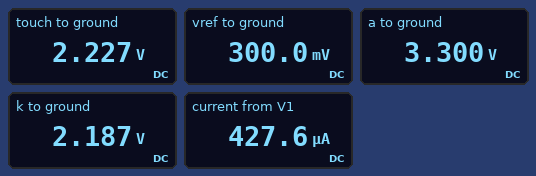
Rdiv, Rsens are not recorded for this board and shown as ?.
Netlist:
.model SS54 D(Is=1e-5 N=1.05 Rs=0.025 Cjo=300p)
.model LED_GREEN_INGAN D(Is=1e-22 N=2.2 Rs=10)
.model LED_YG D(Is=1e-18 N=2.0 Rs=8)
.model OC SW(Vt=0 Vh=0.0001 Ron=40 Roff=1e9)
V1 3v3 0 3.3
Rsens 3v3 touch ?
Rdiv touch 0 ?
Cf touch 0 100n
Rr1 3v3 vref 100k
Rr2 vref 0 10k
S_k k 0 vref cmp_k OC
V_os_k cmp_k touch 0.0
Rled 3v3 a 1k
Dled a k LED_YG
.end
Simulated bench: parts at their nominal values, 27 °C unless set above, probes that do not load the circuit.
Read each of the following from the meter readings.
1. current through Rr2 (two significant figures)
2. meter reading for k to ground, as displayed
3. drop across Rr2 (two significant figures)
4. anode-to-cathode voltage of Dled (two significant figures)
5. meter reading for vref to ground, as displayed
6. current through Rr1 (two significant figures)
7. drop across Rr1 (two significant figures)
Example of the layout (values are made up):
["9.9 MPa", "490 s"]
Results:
["30 µA", "2.187 V", "300 mV", "1.1 V", "300.0 mV", "30 µA", "3.0 V"]
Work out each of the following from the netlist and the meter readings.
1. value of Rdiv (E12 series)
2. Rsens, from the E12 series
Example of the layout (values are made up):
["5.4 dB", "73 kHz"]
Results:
["5.6 kΩ", "2.7 kΩ"]
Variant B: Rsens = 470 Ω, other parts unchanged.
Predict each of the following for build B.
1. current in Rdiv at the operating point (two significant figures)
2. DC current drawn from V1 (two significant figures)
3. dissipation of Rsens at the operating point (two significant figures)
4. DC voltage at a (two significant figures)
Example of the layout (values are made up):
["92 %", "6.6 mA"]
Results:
["540 µA", "570 µA", "140 µW", "3.3 V"]
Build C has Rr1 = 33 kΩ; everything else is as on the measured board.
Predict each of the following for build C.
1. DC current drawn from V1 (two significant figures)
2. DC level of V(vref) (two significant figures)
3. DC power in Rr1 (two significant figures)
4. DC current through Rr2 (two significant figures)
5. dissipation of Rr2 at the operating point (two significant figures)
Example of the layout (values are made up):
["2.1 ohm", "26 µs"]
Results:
["470 µA", "770 mV", "190 µW", "77 µA", "59 µW"]
